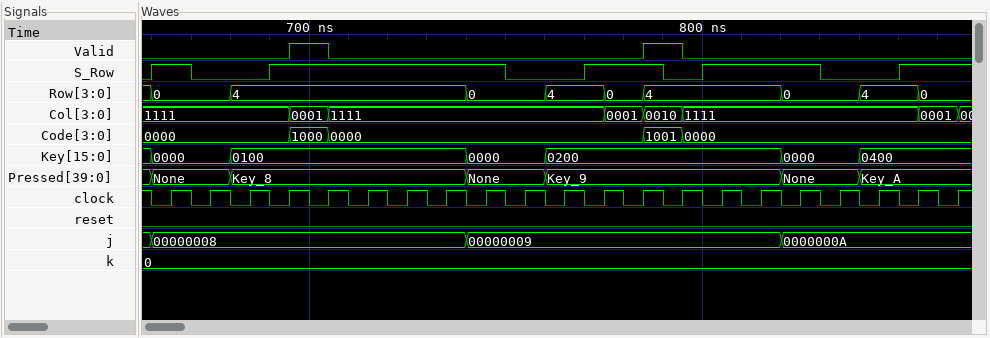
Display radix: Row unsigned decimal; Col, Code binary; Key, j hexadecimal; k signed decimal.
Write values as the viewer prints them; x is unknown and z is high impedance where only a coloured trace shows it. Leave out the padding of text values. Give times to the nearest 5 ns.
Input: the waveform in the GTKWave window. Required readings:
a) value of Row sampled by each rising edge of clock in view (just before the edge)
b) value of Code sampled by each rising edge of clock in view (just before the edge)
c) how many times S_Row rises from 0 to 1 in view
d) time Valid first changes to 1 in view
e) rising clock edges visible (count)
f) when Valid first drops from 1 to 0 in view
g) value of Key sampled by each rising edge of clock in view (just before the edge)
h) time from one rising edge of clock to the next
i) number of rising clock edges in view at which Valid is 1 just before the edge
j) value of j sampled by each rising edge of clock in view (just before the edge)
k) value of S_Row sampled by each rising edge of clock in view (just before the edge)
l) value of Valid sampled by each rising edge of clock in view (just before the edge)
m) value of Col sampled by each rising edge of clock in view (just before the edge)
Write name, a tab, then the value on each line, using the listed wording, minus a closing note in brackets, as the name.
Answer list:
value of Row sampled by each rising edge of clock in view	0, 0, 4, 4, 4, 4, 4, 4, 0, 0, 4, 4, 0, 4, 4, 4, 0, 0, 4, 4, 0
value of Code sampled by each rising edge of clock in view	0000, 0000, 0000, 0000, 1000, 0000, 0000, 0000, 0000, 0000, 0000, 0000, 0000, 1001, 0000, 0000, 0000, 0000, 0000, 0000, 0000
how many times S_Row rises from 0 to 1 in view	5
time Valid first changes to 1 in view	695 ns
rising clock edges visible	21
when Valid first drops from 1 to 0 in view	705 ns
value of Key sampled by each rising edge of clock in view	0000, 0000, 0100, 0100, 0100, 0100, 0100, 0100, 0000, 0000, 0200, 0200, 0200, 0200, 0200, 0200, 0000, 0000, 0400, 0400, 0400
time from one rising edge of clock to the next	10 ns
number of rising clock edges in view at which Valid is 1 just before the edge	2
value of j sampled by each rising edge of clock in view	00000008, 00000008, 00000008, 00000008, 00000008, 00000008, 00000008, 00000008, 00000009, 00000009, 00000009, 00000009, 00000009, 00000009, 00000009, 00000009, 0000000A, 0000000A, 0000000A, 0000000A, 0000000A
value of S_Row sampled by each rising edge of clock in view	1 0 0 1 1 1 1 1 1 0 0 1 1 0 1 1 1 0 0 1 1
value of Valid sampled by each rising edge of clock in view	0 0 0 0 1 0 0 0 0 0 0 0 0 1 0 0 0 0 0 0 0
value of Col sampled by each rising edge of clock in view	1111, 1111, 1111, 1111, 0001, 1111, 1111, 1111, 1111, 1111, 1111, 1111, 0001, 0010, 1111, 1111, 1111, 1111, 1111, 1111, 0001
